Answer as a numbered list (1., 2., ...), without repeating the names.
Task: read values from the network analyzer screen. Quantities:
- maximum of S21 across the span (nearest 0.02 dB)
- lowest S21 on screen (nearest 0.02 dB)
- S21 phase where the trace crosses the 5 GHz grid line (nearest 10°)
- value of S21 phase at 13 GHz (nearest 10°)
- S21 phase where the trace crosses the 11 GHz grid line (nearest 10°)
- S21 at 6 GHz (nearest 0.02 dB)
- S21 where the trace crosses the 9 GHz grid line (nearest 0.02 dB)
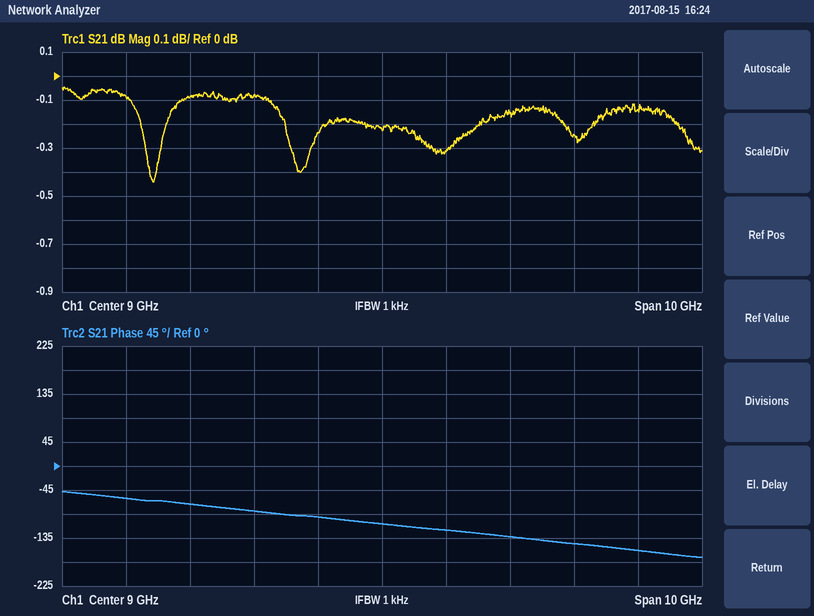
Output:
1. -0.04 dB
2. -0.44 dB
3. -60°
4. -160°
5. -130°
6. -0.08 dB
7. -0.22 dB
